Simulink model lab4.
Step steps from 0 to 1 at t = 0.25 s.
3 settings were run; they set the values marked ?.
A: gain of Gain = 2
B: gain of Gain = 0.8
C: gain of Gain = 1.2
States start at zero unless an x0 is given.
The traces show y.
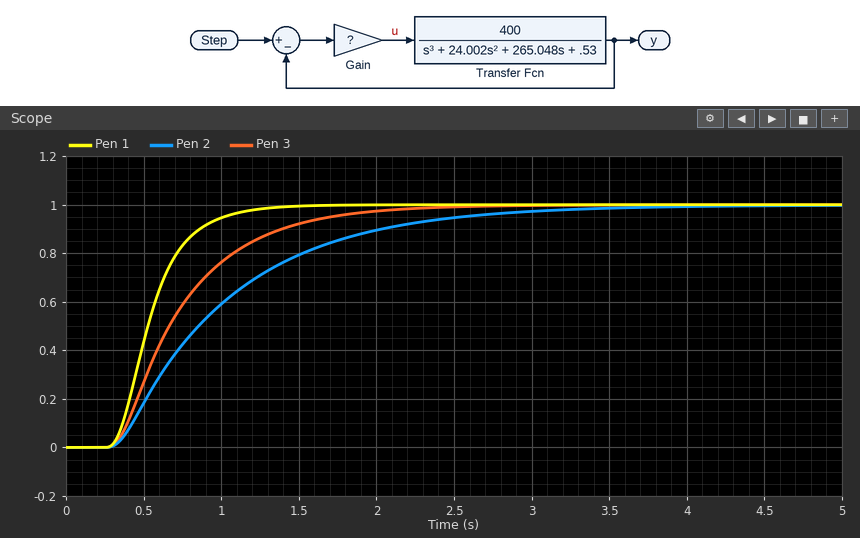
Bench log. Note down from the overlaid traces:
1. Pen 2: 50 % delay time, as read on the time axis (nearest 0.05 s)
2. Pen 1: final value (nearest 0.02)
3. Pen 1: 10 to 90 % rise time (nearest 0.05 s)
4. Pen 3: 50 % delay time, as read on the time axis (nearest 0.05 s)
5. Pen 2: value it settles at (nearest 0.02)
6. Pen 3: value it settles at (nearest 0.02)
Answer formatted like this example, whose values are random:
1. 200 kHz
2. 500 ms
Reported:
1. 0.85 s
2. 1.00
3. 0.50 s
4. 0.65 s
5. 1.00
6. 1.00
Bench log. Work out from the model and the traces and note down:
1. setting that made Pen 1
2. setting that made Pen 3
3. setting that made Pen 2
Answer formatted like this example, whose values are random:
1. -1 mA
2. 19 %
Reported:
1. A
2. C
3. B
